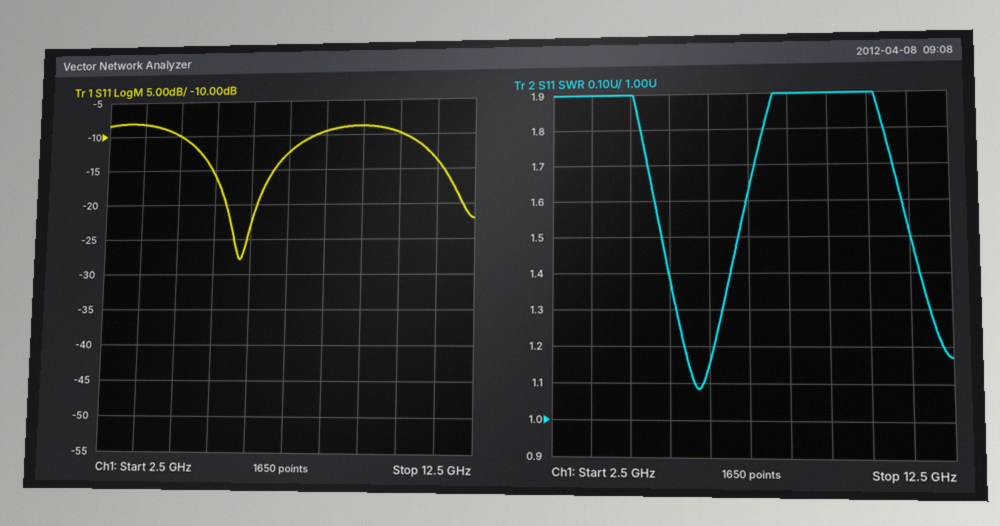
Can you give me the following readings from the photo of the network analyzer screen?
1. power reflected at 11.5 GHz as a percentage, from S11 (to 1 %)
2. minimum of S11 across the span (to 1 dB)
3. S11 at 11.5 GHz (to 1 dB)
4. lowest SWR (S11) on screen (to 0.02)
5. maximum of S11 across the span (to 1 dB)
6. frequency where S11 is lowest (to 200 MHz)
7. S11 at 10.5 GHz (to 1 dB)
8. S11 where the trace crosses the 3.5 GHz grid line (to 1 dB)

4 %
-28 dB
-14 dB
1.08
-8 dB
6.2 GHz
-10 dB
-8 dB
